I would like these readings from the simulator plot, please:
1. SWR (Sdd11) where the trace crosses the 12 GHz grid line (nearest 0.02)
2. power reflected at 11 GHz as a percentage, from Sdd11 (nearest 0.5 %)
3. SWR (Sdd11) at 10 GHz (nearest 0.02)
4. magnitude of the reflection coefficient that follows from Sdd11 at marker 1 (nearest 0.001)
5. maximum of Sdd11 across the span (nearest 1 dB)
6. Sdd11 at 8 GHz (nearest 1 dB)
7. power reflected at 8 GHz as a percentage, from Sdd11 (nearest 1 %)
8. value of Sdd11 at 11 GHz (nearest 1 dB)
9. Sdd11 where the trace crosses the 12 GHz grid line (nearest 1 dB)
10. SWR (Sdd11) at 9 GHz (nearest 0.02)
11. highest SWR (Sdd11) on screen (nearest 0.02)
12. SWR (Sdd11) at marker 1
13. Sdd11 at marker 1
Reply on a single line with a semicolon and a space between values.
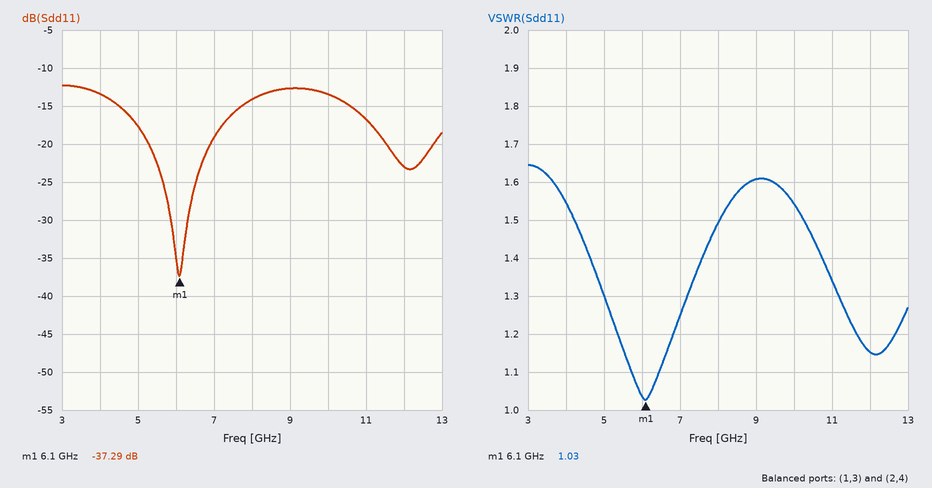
1.16; 2.0 %; 1.54; 0.014; -12 dB; -14 dB; 4 %; -17 dB; -23 dB; 1.60; 1.64; 1.03; -37.29 dB
